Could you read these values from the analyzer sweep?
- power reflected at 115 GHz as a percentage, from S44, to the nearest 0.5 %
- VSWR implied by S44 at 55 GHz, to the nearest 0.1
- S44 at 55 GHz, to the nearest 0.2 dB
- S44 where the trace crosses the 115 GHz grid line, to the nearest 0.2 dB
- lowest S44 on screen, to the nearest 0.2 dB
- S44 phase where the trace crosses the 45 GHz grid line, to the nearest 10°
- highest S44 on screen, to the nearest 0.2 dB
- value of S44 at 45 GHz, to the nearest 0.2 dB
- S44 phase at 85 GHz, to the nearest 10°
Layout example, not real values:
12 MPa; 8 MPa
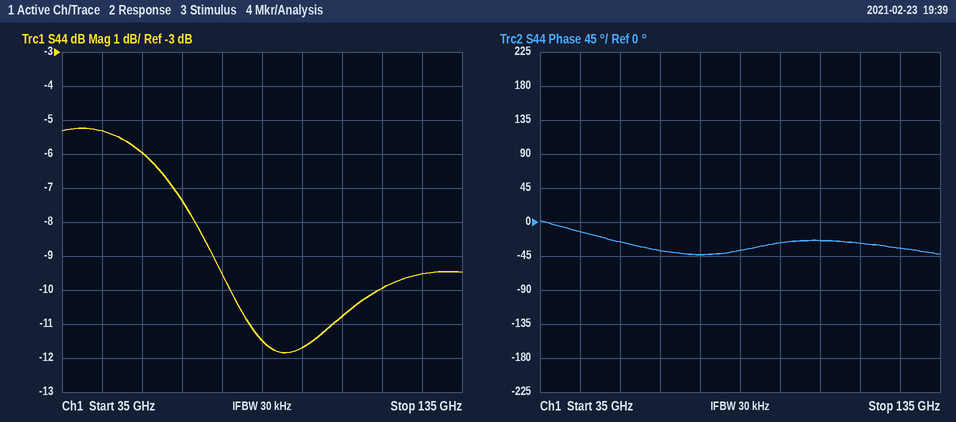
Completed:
10.0 %; 3.0; -6.0 dB; -10.0 dB; -11.8 dB; -10°; -5.2 dB; -5.4 dB; -40°
